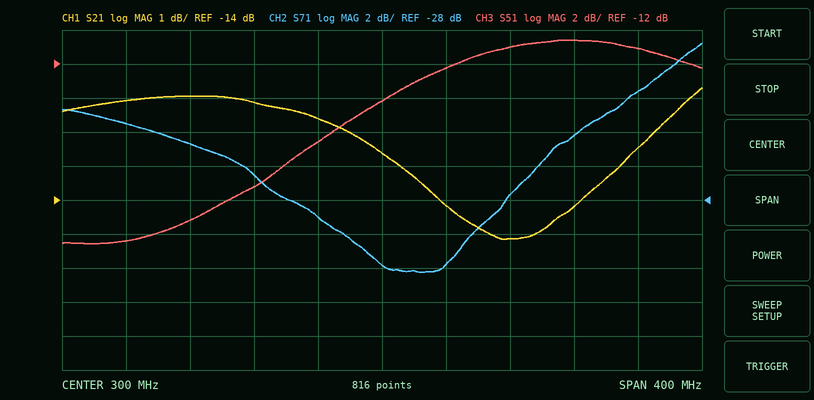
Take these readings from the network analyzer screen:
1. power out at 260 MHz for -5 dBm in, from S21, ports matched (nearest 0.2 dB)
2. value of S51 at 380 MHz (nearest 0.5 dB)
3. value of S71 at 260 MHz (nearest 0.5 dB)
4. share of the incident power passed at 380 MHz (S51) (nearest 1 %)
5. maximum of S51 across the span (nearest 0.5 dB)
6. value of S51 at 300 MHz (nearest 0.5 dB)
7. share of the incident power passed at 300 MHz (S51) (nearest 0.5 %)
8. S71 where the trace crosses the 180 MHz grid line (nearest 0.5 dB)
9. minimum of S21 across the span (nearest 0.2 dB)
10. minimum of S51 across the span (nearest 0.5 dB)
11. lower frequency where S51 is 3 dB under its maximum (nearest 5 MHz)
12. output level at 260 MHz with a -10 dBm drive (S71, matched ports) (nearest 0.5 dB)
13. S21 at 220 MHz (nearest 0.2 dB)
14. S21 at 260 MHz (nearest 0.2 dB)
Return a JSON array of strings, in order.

["-16.6 dBm", "-11.0 dB", "-29.0 dB", "8 %", "-10.5 dB", "-14.0 dB", "4.0 %", "-24.5 dB", "-15.2 dB", "-22.5 dB", "310 MHz", "-39.0 dBm", "-11.2 dB", "-11.6 dB"]
